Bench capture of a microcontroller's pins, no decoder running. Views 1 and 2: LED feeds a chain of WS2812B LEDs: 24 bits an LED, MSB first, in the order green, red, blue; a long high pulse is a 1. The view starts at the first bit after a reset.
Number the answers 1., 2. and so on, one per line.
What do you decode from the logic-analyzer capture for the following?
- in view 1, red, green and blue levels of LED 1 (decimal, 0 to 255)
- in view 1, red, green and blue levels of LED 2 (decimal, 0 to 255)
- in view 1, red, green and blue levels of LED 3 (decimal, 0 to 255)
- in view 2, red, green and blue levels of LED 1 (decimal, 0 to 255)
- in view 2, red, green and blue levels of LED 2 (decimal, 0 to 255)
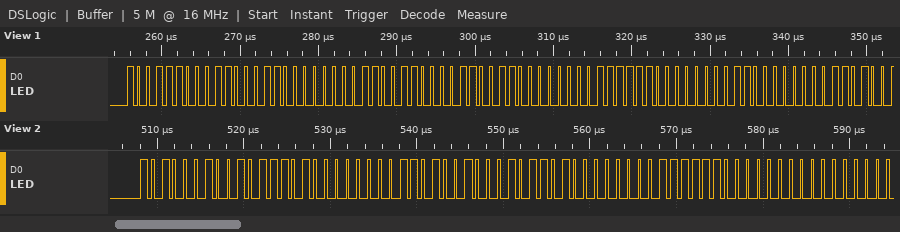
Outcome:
1. 99, 156, 0
2. 51, 204, 0
3. 3, 252, 0
4. 93, 162, 0
5. 45, 210, 0
